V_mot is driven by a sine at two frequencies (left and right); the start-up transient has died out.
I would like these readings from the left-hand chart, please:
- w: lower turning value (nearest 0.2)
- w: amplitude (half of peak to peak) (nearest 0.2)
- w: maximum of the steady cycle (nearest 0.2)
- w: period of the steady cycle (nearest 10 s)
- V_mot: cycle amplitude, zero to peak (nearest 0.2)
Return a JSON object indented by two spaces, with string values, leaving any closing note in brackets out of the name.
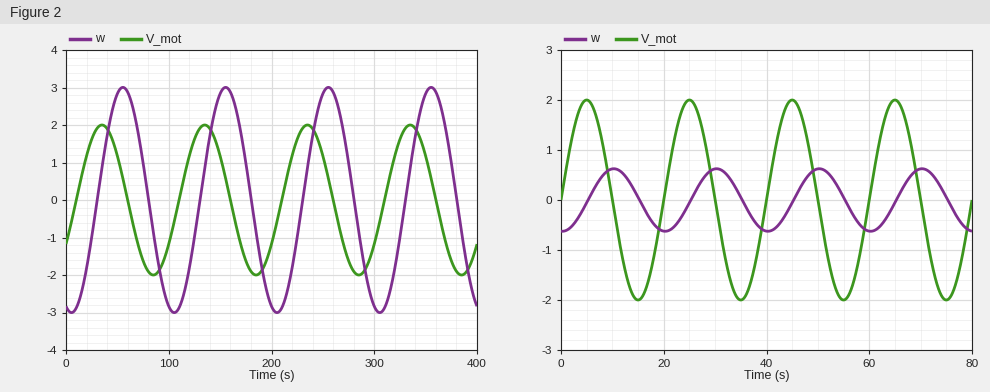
{
  "w: lower turning value": "-3.0",
  "w: amplitude (half of peak to peak)": "3.0",
  "w: maximum of the steady cycle": "3.0",
  "w: period of the steady cycle": "100 s",
  "V_mot: cycle amplitude, zero to peak": "2.0"
}
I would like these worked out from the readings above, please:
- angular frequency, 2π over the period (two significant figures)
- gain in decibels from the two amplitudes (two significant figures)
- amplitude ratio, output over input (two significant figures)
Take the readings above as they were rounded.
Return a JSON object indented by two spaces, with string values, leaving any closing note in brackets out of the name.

{
  "angular frequency, 2π over the period": "0.063 rad/s",
  "gain in decibels from the two amplitudes": "3.5 dB",
  "amplitude ratio, output over input": "1.5"
}
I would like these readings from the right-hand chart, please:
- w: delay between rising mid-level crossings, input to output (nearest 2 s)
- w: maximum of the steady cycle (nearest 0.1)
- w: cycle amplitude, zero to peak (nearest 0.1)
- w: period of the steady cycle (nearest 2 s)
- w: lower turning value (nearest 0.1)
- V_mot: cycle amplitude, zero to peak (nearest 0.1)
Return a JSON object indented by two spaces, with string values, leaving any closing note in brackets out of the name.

{
  "w: delay between rising mid-level crossings, input to output": "6 s",
  "w: maximum of the steady cycle": "0.6",
  "w: cycle amplitude, zero to peak": "0.6",
  "w: period of the steady cycle": "20 s",
  "w: lower turning value": "-0.6",
  "V_mot: cycle amplitude, zero to peak": "2.0"
}
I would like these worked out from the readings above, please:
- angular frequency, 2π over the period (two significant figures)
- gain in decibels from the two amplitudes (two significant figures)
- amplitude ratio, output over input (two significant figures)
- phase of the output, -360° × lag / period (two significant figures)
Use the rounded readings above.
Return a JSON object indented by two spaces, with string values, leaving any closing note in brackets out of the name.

{
  "angular frequency, 2π over the period": "0.31 rad/s",
  "gain in decibels from the two amplitudes": "-10 dB",
  "amplitude ratio, output over input": "0.30",
  "phase of the output, -360° × lag / period": "-110°"
}
